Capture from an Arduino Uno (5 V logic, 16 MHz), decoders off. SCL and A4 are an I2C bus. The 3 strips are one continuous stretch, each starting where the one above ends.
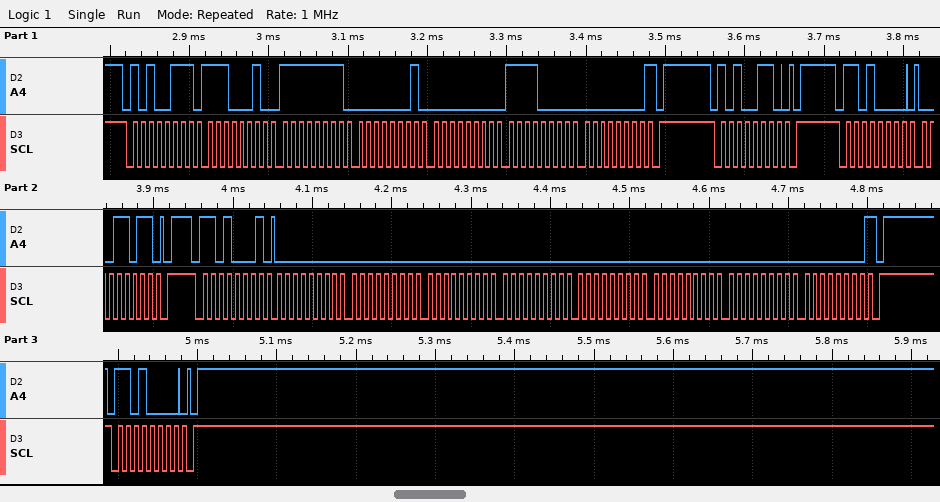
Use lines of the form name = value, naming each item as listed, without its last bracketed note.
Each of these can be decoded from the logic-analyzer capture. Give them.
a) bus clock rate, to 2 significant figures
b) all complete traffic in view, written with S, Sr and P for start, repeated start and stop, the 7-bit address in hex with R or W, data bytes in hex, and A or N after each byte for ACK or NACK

bus clock rate, to 2 significant figures = 100 kHz
all complete traffic in view, written with S, Sr and P for start, repeated start and stop, the 7-bit address in hex with R or W, data bytes in hex, and A or N after each byte for ACK or NACK = S 53R A E2 A FF A 01 A 00 A F0 A 00 N P S 53W A P S 68W A 1B A P S 68R A 00 A 00 A 00 A 00 A 00 A 00 A 00 A 00 N P S 68W A P
